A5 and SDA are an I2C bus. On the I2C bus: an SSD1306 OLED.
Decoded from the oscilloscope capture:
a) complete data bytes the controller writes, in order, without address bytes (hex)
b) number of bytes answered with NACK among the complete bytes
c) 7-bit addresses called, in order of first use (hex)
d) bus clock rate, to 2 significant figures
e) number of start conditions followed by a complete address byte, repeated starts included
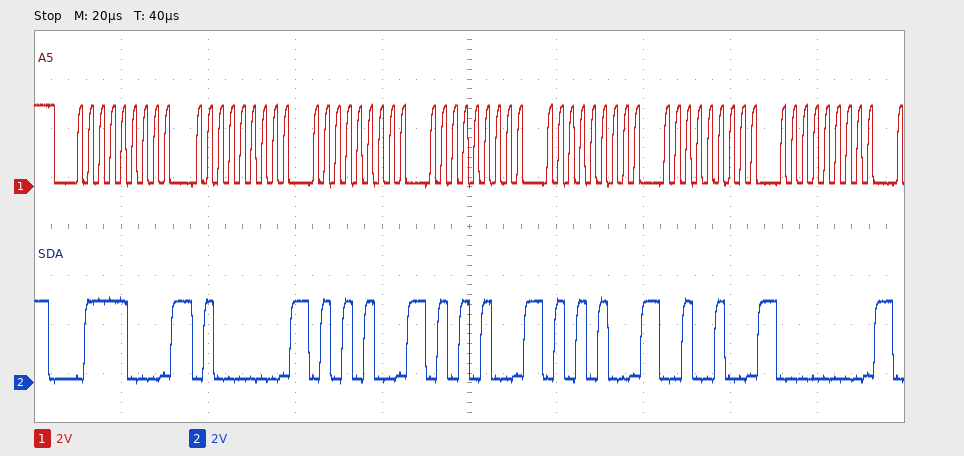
40 54 54 54 24 00
0
0x3C
400 kHz
1
